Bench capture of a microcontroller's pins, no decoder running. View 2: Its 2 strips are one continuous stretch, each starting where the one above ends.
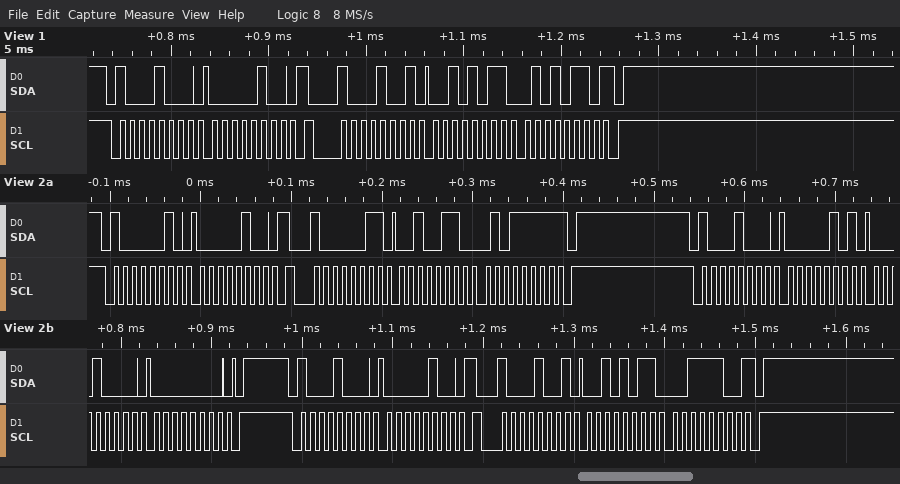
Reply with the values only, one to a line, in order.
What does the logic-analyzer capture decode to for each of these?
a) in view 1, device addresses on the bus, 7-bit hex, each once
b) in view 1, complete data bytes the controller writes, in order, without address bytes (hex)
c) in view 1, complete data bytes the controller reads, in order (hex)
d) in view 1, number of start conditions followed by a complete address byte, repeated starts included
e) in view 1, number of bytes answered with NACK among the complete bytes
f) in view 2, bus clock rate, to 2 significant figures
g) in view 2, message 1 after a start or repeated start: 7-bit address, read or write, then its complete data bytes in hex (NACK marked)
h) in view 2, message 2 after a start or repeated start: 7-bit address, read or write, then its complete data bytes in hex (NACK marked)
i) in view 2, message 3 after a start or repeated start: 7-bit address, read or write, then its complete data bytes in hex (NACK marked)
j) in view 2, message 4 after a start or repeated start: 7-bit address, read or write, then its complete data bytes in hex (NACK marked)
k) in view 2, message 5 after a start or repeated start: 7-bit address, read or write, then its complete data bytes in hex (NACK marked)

0x44
04
2B 56
2
1
100 kHz
0x41 write: 04
0x41 read: 26 5F NACK
0x44 write: 05 10 00
0x44 write: 04
0x44 read: 2B 3C NACK
